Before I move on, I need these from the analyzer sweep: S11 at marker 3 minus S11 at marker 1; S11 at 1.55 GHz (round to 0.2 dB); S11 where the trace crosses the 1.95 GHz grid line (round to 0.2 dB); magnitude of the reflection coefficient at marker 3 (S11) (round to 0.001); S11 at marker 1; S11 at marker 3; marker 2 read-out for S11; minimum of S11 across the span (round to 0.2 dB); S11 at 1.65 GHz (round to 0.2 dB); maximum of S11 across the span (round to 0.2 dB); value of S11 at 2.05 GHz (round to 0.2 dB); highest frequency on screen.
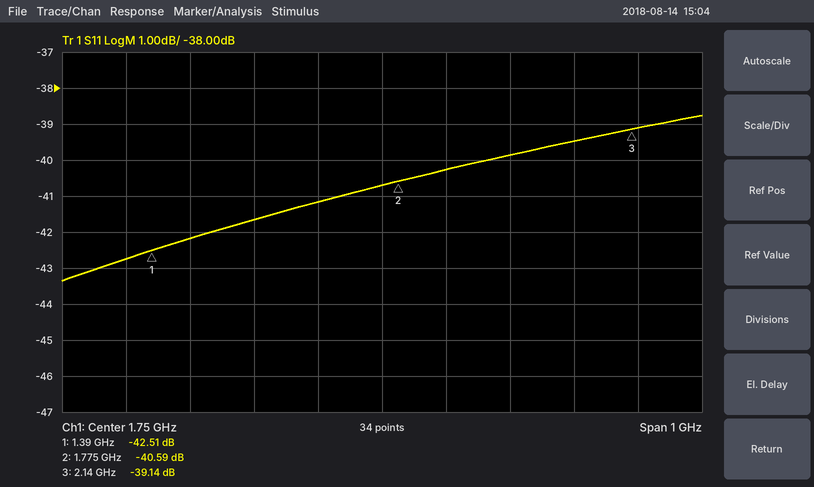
3.37 dB
-41.6 dB
-39.8 dB
0.011
-42.51 dB
-39.14 dB
-40.59 dB
-43.4 dB
-41.2 dB
-38.8 dB
-39.4 dB
2.25 GHz
